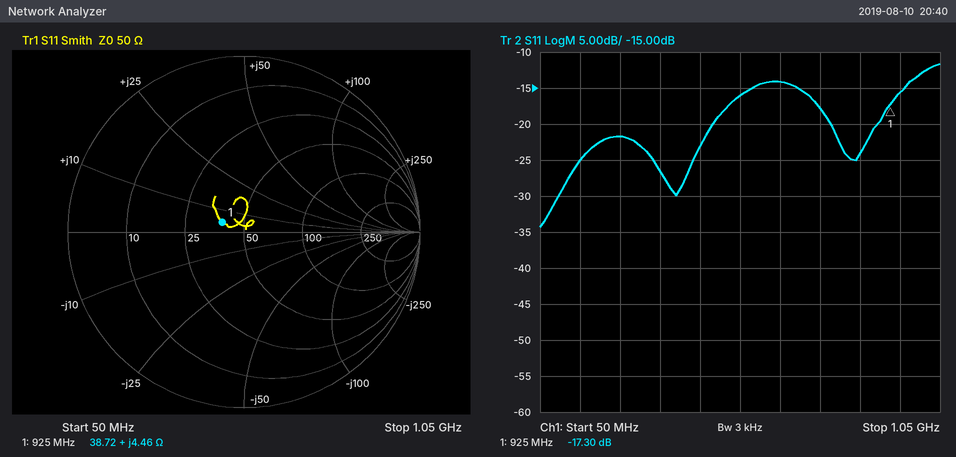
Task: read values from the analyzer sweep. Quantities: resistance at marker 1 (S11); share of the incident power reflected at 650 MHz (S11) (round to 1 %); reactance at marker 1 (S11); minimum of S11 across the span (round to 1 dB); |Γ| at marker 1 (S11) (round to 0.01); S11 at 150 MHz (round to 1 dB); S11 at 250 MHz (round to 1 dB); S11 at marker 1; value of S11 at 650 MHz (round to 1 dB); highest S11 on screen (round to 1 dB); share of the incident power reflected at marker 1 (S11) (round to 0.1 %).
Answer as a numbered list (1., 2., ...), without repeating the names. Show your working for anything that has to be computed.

1. 38.72 Ω
2. 10^(-14/10) ≈ 4 %
3. +4.46 Ω
4. -34 dB
5. 0.14
6. -25 dB
7. -22 dB
8. -17.30 dB
9. -14 dB
10. -12 dB
11. 10^(-17.3/10) ≈ 1.9 %
